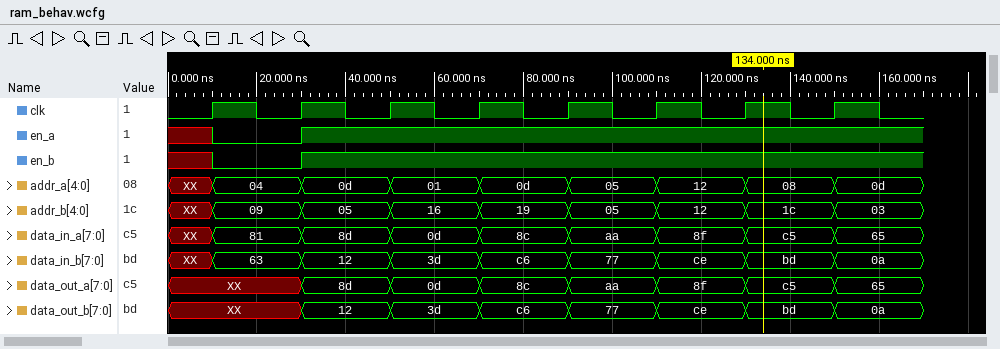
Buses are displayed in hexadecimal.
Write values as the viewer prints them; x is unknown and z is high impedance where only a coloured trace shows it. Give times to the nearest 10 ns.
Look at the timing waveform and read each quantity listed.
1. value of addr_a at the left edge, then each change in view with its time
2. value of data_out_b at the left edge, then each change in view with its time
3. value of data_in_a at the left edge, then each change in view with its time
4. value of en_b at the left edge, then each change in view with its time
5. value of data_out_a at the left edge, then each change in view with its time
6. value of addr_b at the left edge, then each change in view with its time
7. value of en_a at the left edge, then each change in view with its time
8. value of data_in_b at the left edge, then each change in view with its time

XX, 04 at 10 ns, 0d at 30 ns, 01 at 50 ns, 0d at 70 ns, 05 at 90 ns, 12 at 110 ns, 08 at 130 ns, 0d at 150 ns
XX, 12 at 30 ns, 3d at 50 ns, c6 at 70 ns, 77 at 90 ns, ce at 110 ns, bd at 130 ns, 0a at 150 ns
XX, 81 at 10 ns, 8d at 30 ns, 0d at 50 ns, 8c at 70 ns, aa at 90 ns, 8f at 110 ns, c5 at 130 ns, 65 at 150 ns
x, 0 at 10 ns, 1 at 30 ns
XX, 8d at 30 ns, 0d at 50 ns, 8c at 70 ns, aa at 90 ns, 8f at 110 ns, c5 at 130 ns, 65 at 150 ns
XX, 09 at 10 ns, 05 at 30 ns, 16 at 50 ns, 19 at 70 ns, 05 at 90 ns, 12 at 110 ns, 1c at 130 ns, 03 at 150 ns
x, 0 at 10 ns, 1 at 30 ns
XX, 63 at 10 ns, 12 at 30 ns, 3d at 50 ns, c6 at 70 ns, 77 at 90 ns, ce at 110 ns, bd at 130 ns, 0a at 150 ns
